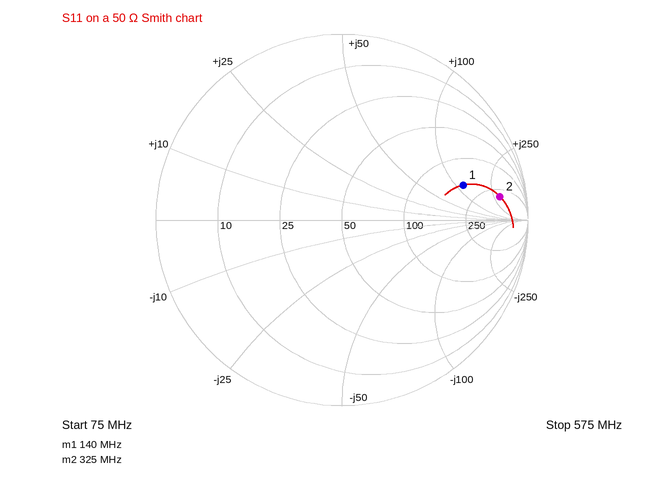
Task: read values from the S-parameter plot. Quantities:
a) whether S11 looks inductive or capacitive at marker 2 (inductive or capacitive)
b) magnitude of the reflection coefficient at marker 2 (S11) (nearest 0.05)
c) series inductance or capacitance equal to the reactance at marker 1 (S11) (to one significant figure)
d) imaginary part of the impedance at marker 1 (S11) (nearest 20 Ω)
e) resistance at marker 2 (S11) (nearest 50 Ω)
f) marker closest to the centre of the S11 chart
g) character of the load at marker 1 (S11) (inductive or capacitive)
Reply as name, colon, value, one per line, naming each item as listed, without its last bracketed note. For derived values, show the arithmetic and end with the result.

whether S11 looks inductive or capacitive at marker 2: inductive
magnitude of the reflection coefficient at marker 2 (S11): 0.85
series inductance or capacitance equal to the reactance at marker 1 (S11): L = 120 Ω/(2π × 140 MHz) ≈ 136 nH, so 100 nH to one significant figure
imaginary part of the impedance at marker 1 (S11): +120 Ω
resistance at marker 2 (S11): 350 Ω
marker closest to the centre of the S11 chart: marker 1
character of the load at marker 1 (S11): inductive
